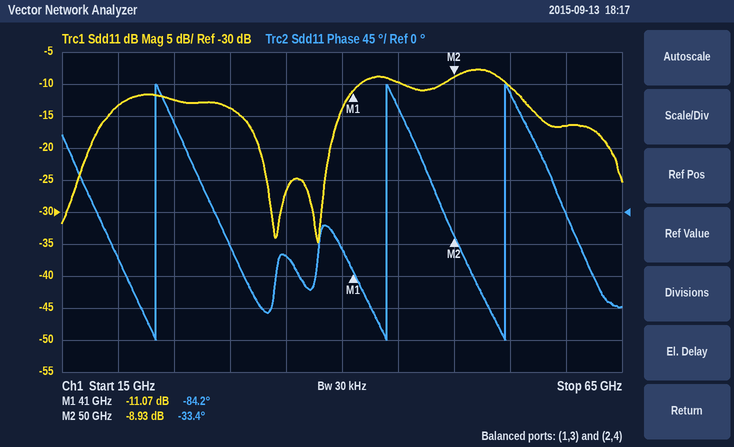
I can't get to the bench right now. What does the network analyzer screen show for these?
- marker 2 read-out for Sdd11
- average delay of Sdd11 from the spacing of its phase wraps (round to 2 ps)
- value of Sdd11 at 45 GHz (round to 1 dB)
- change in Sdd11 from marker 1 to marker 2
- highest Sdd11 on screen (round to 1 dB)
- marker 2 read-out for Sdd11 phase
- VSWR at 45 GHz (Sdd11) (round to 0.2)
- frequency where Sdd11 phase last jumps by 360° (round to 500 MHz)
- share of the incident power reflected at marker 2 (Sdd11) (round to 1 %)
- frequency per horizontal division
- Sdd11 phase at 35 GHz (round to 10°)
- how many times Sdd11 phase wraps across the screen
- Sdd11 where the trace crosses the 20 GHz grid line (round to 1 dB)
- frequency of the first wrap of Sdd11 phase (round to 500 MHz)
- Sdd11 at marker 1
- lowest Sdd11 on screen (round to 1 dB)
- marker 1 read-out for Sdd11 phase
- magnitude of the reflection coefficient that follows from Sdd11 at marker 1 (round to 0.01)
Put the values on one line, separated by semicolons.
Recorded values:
-8.93 dB; 64 ps; -10 dB; 2.14 dB; -8 dB; -33.4°; 2.0; 54.5 GHz; 13 %; 5 GHz; -60°; 3; -13 dB; 23.5 GHz; -11.07 dB; -35 dB; -84.2°; 0.28
